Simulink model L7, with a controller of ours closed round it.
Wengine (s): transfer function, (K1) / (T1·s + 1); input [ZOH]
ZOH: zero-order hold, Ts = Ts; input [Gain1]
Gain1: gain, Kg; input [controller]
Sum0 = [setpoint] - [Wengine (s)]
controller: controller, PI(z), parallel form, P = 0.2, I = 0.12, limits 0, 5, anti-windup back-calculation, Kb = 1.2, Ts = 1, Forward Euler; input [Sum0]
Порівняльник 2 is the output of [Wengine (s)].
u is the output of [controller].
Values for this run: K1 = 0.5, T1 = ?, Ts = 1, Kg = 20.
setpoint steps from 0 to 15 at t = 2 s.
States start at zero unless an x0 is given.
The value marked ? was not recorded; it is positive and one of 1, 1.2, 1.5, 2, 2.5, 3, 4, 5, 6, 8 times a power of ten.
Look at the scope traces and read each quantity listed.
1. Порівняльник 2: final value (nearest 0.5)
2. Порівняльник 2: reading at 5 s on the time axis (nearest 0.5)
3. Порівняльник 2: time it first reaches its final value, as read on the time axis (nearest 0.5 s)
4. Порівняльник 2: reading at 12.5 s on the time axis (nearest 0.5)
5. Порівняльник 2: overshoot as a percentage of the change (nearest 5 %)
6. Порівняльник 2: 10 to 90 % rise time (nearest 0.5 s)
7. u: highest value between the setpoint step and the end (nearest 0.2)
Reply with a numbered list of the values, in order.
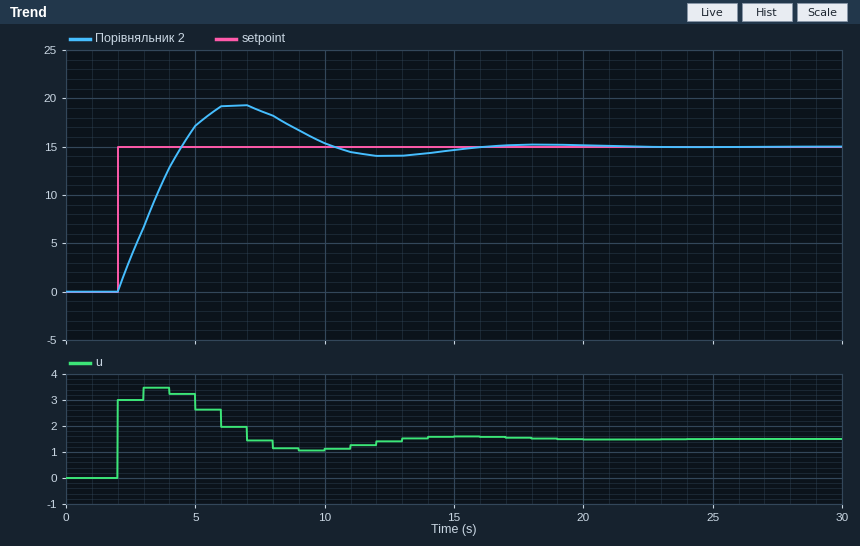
1. 15.0
2. 17.0
3. 4.5 s
4. 14.0
5. 30 %
6. 2.0 s
7. 3.4
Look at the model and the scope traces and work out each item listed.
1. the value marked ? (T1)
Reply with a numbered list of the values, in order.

1. 4
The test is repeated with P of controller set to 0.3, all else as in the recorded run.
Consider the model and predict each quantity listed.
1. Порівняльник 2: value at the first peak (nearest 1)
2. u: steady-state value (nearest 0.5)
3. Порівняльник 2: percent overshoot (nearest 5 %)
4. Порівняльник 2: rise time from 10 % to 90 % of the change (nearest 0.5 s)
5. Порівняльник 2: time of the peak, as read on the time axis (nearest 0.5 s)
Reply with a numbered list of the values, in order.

1. 17
2. 1.5
3. 15 %
4. 1.5 s
5. 6.0 s
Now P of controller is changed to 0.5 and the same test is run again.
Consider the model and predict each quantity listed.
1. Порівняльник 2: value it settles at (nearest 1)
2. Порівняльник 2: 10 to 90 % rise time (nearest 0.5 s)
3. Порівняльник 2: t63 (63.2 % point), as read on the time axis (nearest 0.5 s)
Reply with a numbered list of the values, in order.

1. 15
2. 6.0 s
3. 3.0 s
